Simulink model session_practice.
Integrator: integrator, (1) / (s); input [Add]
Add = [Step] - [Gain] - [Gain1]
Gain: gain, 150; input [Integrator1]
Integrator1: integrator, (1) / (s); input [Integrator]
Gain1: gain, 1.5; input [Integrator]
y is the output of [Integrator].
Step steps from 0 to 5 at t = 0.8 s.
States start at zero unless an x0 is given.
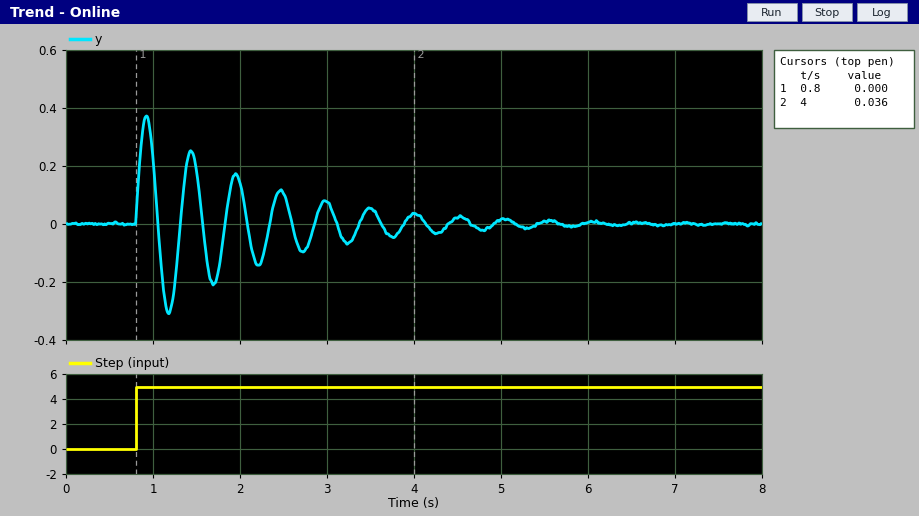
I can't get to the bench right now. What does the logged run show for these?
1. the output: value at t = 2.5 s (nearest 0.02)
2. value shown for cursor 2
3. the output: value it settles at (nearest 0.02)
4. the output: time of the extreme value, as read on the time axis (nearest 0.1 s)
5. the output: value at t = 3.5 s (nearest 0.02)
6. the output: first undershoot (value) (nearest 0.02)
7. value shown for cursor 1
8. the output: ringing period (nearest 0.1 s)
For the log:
0.10
0.036
0.00
0.9 s
0.06
-0.30
0.000
0.5 s
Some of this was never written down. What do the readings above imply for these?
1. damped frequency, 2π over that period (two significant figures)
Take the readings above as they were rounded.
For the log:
13 rad/s
